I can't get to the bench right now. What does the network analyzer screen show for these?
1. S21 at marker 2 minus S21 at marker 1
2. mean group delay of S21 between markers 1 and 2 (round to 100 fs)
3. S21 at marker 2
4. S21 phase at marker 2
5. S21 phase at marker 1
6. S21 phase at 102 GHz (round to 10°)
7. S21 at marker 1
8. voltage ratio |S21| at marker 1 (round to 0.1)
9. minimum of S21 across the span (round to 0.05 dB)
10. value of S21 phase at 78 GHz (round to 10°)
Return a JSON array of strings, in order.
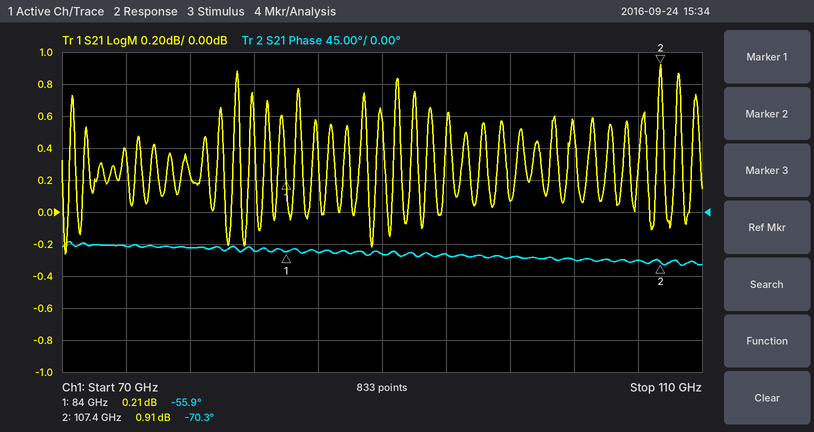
["0.70 dB", "1.7 ps", "0.91 dB", "-70.3°", "-55.9°", "-70°", "0.21 dB", "1.0", "-0.25 dB", "-50°"]
